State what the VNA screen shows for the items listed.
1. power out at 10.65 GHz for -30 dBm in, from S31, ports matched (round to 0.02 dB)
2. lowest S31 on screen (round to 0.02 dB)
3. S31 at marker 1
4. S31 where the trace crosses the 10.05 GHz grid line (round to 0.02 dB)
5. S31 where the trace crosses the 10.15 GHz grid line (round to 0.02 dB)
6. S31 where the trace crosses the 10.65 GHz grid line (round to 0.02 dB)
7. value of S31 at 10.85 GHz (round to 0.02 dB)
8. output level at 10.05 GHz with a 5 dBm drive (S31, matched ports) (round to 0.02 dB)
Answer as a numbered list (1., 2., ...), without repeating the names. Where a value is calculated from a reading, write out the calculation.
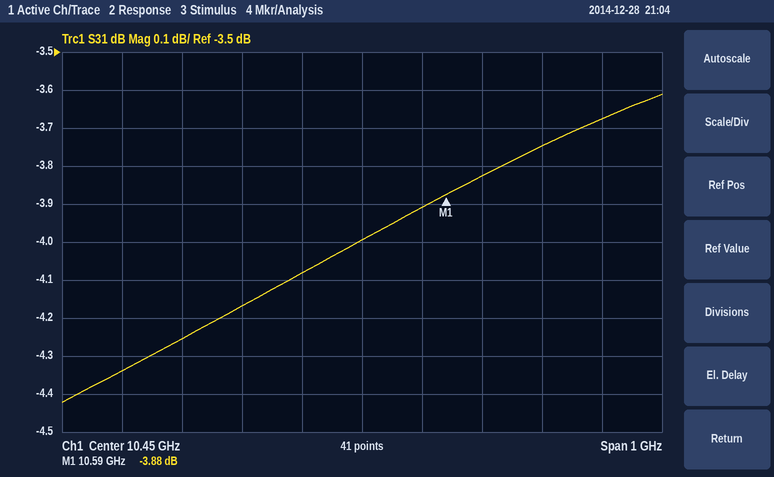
1. -30 dBm + (-3.82 dB) = -33.82 dBm
2. -4.42 dB
3. -3.88 dB
4. -4.34 dB
5. -4.26 dB
6. -3.82 dB
7. -3.68 dB
8. 5 dBm + (-4.34 dB) = 0.66 dBm
